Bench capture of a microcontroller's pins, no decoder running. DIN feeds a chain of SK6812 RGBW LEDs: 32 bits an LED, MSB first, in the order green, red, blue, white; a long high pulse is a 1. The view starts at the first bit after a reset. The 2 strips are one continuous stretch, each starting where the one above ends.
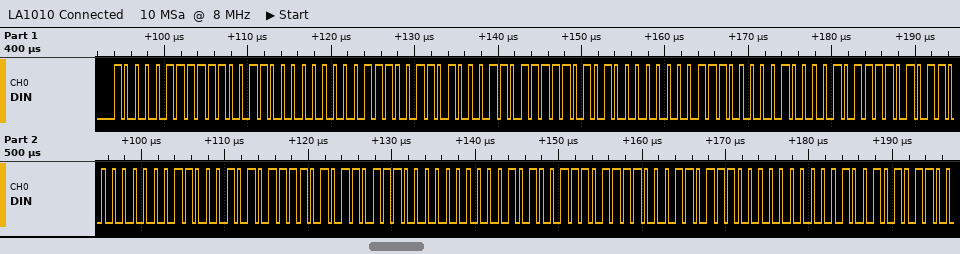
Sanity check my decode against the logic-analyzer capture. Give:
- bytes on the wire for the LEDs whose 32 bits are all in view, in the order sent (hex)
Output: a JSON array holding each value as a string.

["87 E6 00 E6 8D F5 00 E0 85 EB 00 C5 7A DC 00 A7 78 DC 00 95"]
